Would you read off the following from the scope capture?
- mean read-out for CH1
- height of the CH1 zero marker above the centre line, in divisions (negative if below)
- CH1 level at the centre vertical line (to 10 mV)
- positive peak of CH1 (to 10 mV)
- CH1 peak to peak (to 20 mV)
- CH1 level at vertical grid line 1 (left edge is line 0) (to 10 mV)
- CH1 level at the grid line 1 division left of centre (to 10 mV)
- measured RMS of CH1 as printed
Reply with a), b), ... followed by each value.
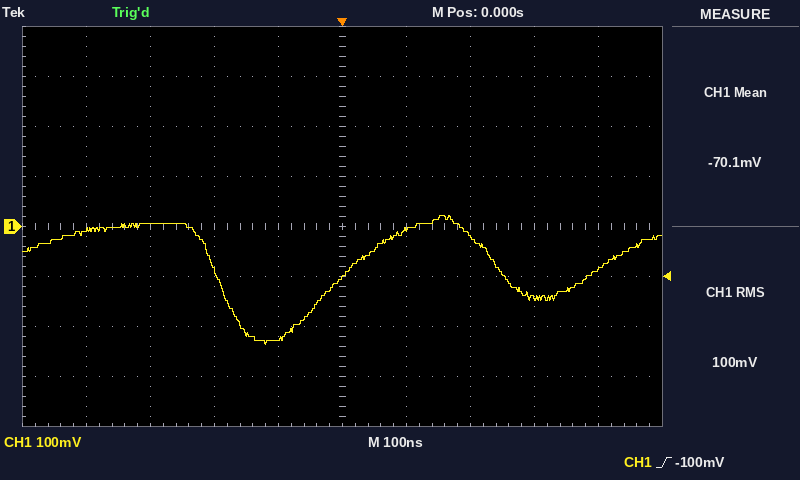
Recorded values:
a) -70.1 mV
b) 0.0 div
c) -100 mV
d) 20 mV
e) 260 mV
f) -10 mV
g) -220 mV
h) 100 mV
